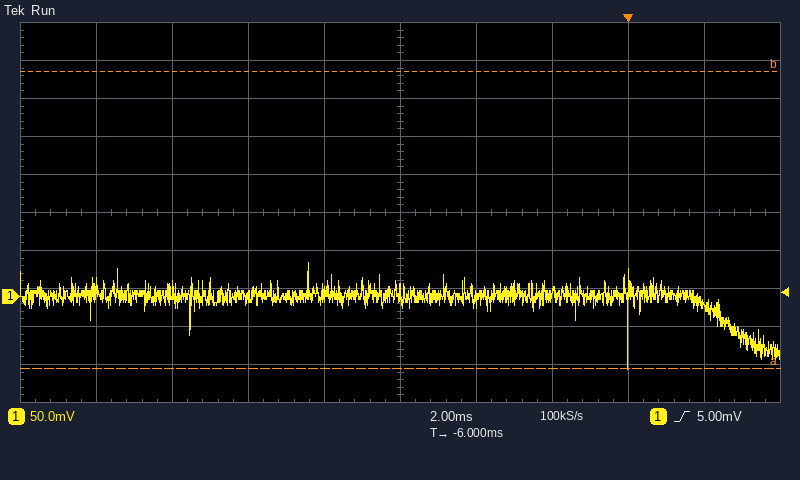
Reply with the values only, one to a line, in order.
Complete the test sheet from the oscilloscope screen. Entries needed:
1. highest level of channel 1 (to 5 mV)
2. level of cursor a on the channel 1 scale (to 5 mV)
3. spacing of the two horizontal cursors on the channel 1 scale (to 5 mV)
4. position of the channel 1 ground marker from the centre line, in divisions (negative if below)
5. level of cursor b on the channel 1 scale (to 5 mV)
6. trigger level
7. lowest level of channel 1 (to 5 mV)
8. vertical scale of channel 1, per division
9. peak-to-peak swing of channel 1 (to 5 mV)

45 mV
-95 mV
390 mV
-2.2 div
295 mV
5.00 mV
-95 mV
50 mV
140 mV
